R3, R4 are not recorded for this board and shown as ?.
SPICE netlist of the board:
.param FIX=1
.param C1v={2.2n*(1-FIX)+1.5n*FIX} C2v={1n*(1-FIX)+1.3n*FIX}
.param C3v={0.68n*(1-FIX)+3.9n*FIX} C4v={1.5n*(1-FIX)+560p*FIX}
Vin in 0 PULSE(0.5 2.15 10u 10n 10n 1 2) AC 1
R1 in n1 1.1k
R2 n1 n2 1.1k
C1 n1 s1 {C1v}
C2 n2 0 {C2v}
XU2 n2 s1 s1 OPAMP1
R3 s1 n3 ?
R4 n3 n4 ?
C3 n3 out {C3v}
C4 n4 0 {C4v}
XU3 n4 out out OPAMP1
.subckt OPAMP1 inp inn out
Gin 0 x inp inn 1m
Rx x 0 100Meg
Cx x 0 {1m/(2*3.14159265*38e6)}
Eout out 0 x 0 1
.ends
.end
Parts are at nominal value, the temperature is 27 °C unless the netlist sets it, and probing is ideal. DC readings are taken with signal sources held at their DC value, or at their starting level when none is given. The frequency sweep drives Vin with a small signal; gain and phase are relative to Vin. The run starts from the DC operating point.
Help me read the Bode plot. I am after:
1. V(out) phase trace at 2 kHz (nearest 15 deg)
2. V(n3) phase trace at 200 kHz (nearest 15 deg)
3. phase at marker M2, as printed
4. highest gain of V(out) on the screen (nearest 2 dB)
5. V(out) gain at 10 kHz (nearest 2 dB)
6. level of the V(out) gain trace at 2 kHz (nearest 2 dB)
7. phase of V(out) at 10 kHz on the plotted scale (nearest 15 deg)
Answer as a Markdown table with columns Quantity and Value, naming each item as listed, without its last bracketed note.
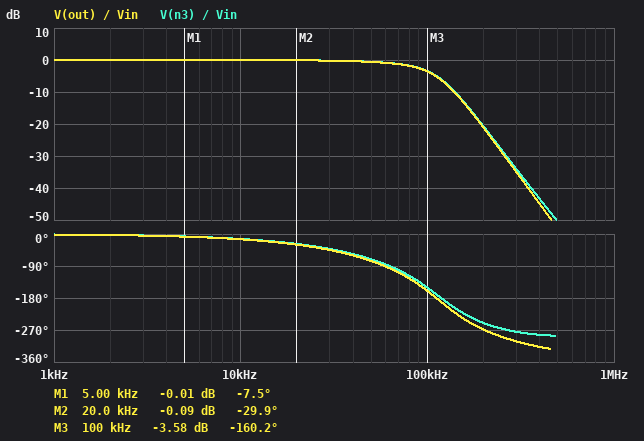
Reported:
| Quantity | Value |
|---|---|
| V(out) phase trace at 2 kHz | 0 deg |
| V(n3) phase trace at 200 kHz | -255 deg |
| phase at marker M2, as printed | -29.9 deg |
| highest gain of V(out) on the screen | 0 dB |
| V(out) gain at 10 kHz | 0 dB |
| level of the V(out) gain trace at 2 kHz | 0 dB |
| phase of V(out) at 10 kHz on the plotted scale | -15 deg |
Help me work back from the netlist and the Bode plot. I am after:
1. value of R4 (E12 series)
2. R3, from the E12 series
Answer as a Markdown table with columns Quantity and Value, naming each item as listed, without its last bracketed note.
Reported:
| Quantity | Value |
|---|---|
| value of R4 | 470 Ω |
| R3, from the E12 series | 1.8 kΩ |
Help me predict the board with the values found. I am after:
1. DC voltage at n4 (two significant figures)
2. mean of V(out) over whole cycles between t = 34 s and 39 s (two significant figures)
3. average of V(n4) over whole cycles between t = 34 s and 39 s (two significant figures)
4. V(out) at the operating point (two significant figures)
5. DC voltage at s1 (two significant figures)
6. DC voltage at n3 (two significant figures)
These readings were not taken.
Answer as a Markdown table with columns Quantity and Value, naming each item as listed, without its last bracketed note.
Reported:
| Quantity | Value |
|---|---|
| DC voltage at n4 | 500 mV |
| mean of V(out) over whole cycles between t = 34 s and 39 s | 1.3 V |
| average of V(n4) over whole cycles between t = 34 s and 39 s | 1.3 V |
| V(out) at the operating point | 500 mV |
| DC voltage at s1 | 500 mV |
| DC voltage at n3 | 500 mV |
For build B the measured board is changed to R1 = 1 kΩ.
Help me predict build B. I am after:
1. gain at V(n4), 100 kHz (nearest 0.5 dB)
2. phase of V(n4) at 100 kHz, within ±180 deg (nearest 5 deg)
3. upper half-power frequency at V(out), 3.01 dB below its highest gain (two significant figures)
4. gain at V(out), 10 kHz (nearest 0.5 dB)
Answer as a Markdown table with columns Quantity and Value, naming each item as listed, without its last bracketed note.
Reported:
| Quantity | Value |
|---|---|
| gain at V(n4), 100 kHz | -3.0 dB |
| phase of V(n4) at 100 kHz, within ±180 deg | -155 deg |
| upper half-power frequency at V(out), 3.01 dB below its highest gain | 98 kHz |
| gain at V(out), 10 kHz | 0 dB |
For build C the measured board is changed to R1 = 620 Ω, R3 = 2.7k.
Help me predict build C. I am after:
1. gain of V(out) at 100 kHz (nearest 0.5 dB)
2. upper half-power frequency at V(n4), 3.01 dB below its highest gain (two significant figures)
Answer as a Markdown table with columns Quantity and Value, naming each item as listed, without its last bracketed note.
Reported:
| Quantity | Value |
|---|---|
| gain of V(out) at 100 kHz | -4.5 dB |
| upper half-power frequency at V(n4), 3.01 dB below its highest gain | 91 kHz |
